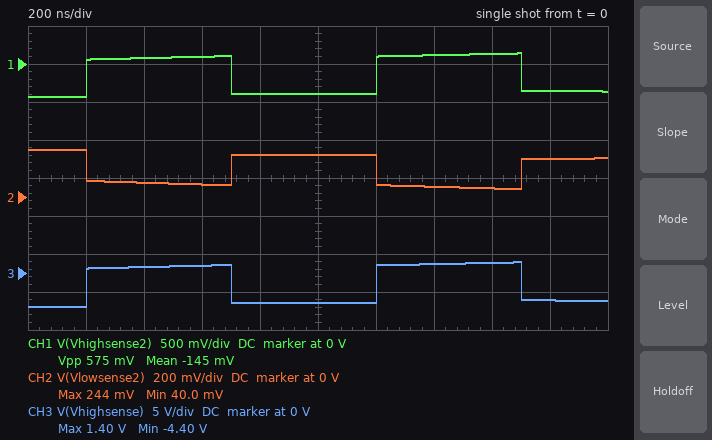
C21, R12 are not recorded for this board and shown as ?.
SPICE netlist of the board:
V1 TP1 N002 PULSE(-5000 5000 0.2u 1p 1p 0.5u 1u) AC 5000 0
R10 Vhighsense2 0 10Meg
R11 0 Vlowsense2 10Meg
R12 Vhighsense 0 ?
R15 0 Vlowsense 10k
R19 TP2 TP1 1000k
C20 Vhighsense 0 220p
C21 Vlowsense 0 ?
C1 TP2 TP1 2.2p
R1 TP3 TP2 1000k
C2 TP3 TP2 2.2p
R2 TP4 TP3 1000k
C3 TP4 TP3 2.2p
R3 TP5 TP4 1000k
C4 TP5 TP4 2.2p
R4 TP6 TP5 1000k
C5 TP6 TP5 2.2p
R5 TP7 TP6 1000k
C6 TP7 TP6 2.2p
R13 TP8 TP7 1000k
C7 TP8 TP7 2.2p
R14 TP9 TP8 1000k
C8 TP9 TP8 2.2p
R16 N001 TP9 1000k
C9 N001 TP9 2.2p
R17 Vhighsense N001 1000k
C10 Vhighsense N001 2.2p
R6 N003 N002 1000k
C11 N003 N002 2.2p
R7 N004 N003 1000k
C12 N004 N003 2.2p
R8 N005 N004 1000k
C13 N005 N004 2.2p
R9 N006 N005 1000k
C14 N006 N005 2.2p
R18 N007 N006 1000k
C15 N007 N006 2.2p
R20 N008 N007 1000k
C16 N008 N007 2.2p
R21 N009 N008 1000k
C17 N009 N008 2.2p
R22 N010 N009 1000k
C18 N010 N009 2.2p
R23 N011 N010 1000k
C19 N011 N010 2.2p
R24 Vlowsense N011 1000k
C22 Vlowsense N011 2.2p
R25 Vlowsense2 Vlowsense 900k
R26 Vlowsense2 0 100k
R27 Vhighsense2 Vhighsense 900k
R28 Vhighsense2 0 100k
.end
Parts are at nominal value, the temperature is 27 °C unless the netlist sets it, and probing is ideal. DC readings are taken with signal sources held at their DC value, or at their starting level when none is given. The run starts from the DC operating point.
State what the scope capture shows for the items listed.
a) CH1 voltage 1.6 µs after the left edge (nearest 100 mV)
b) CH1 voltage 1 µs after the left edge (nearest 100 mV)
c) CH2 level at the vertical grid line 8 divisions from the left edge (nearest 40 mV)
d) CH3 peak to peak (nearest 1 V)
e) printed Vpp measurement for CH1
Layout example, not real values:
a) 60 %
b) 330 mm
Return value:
a) 100 mV
b) -400 mV
c) 40 mV
d) 6 V
e) 575 mV
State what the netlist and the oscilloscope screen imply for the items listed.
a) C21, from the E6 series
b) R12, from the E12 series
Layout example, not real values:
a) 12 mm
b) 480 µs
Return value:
a) 680 pF
b) 18 kΩ
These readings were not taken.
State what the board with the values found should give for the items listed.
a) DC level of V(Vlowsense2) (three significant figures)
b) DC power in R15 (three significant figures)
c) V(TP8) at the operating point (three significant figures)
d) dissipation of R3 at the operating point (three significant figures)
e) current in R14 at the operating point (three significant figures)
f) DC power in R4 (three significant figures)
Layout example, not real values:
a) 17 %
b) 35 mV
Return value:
a) 245 mV
b) 611 µW
c) -753 V
d) 62.3 mW
e) 250 µA
f) 62.3 mW
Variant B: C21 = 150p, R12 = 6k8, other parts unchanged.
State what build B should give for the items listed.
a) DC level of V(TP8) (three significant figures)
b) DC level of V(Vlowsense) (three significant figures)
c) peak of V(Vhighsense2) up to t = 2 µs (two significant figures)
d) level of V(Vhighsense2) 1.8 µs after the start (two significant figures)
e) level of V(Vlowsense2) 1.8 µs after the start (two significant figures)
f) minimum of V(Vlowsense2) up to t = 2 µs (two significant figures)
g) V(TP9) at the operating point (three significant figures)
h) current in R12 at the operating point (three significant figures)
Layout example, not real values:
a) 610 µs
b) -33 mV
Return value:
a) -751 V
b) 2.47 V
c) 330 mV
d) -230 mV
e) 340 mV
f) -480 mV
g) -501 V
h) 248 µA
